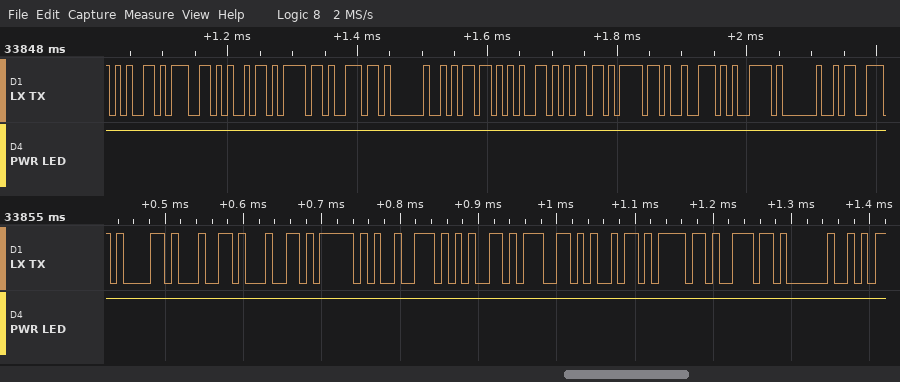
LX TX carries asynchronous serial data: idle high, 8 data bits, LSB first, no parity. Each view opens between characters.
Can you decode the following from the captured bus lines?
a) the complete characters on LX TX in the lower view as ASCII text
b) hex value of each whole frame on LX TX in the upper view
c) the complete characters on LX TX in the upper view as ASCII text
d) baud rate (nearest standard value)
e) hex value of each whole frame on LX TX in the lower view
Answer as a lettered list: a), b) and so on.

a) "add_region "
b) 65, 67, 69, 6F, 6E, 20, 6D, 65, 6D, 6F, 72, 79, 20
c) "egion memory "
d) 115200 baud
e) 61, 64, 64, 5F, 72, 65, 67, 69, 6F, 6E, 20
